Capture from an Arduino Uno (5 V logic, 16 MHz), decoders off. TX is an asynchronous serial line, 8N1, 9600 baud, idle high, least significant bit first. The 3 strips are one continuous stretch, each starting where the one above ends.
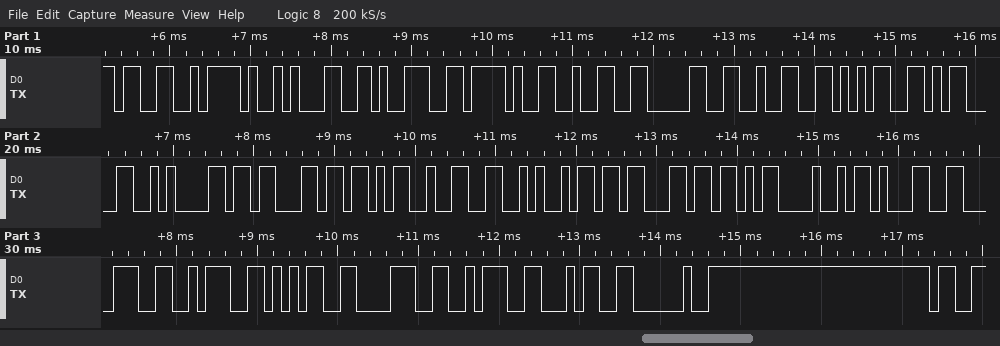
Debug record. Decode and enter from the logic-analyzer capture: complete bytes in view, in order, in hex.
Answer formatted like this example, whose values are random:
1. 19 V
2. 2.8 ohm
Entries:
1. 33 2F 31 39 2F 32 30 32 35 0D 0A 1B 5B 32 4A 1B 5B 48 31 38 3A 35 38 3A 34 20
